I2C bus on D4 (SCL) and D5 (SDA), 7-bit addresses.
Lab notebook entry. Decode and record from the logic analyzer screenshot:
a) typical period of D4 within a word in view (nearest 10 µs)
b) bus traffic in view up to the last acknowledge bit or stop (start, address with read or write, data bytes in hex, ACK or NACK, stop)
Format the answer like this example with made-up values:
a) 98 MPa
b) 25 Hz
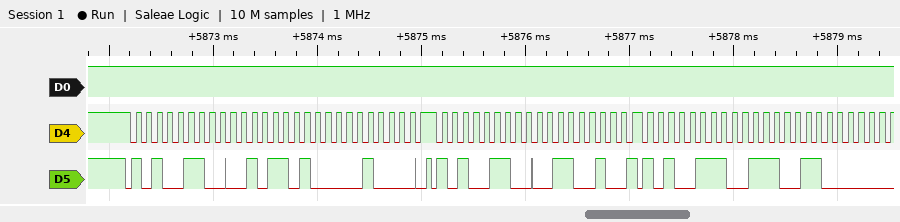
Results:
a) 100 µs
b) start, address 53 write ACK, 2D ACK, 08 ACK, stop, start, address 53 write ACK, 32 ACK, repeated start, address 53 read ACK, 73 ACK
